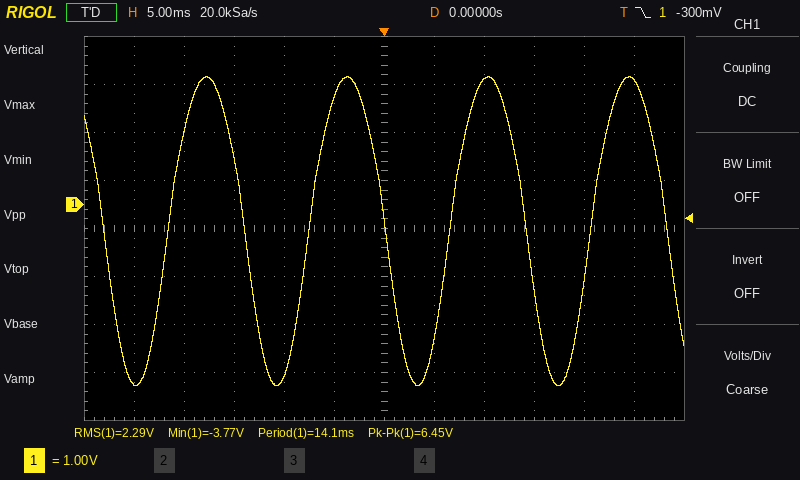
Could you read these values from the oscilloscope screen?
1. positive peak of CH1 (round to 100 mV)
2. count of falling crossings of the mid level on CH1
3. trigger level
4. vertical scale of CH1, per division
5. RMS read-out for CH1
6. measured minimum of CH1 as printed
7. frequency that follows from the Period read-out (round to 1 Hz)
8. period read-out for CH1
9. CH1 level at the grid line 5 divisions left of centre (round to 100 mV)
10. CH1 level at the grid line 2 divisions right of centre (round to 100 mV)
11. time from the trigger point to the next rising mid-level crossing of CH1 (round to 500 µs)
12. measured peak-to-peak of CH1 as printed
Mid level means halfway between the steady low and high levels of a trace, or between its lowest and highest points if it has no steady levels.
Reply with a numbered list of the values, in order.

1. 2.7 V
2. 5
3. -300 mV
4. 1 V
5. 2.29 V
6. -3.77 V
7. 71 Hz
8. 14.1 ms
9. -3.7 V
10. 2.6 V
11. 6.5 ms
12. 6.45 V
